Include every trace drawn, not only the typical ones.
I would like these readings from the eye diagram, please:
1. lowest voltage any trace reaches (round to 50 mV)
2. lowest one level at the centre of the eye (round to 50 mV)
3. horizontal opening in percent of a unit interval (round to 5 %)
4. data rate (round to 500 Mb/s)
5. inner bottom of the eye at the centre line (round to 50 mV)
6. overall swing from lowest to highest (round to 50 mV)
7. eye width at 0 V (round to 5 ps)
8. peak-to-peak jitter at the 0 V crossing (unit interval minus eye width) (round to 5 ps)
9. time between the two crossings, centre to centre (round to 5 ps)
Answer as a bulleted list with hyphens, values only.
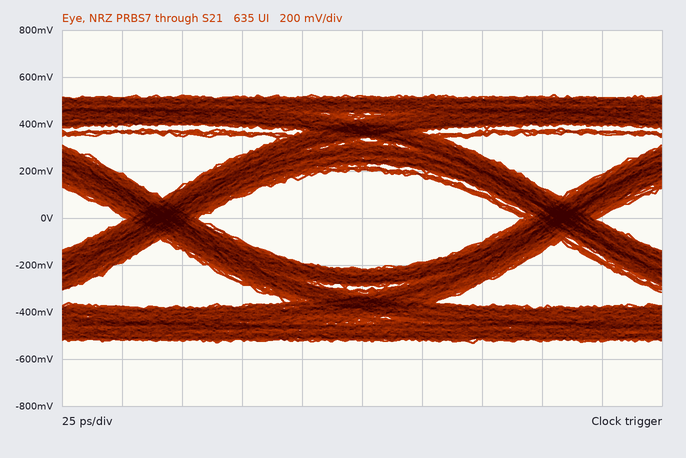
- -550 mV
- 200 mV
- 80 %
- 6.0 Gb/s
- -200 mV
- 1.05 V
- 135 ps
- 30 ps
- 165 ps
